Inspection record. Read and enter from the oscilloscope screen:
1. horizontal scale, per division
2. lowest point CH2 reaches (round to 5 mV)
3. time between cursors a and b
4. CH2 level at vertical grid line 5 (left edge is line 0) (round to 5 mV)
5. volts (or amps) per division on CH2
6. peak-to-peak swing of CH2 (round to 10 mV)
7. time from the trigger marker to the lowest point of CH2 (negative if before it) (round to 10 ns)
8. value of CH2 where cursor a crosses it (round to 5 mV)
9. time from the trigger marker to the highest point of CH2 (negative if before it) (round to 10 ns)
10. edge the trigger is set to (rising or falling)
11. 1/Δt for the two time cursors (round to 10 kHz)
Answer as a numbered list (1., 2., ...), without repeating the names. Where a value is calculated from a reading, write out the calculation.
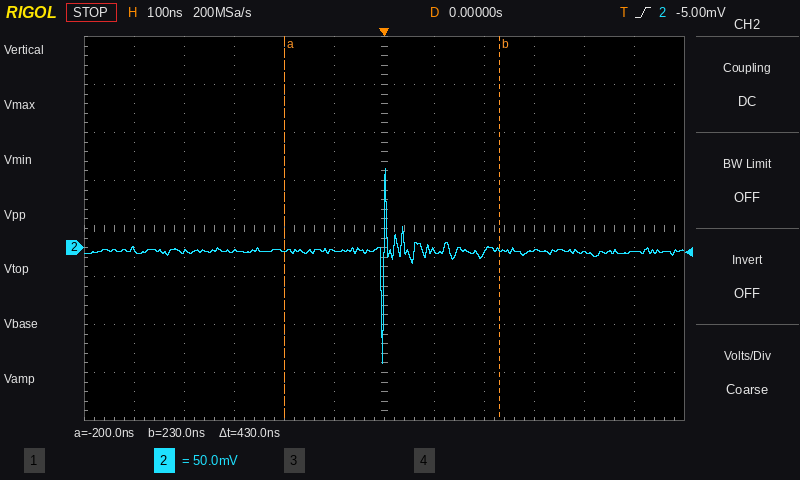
1. 100 ns
2. -120 mV
3. 430 ns
4. -5 mV
5. 50 mV
6. 200 mV
7. 0 ns
8. -5 mV
9. 0 ns
10. rising
11. 1 / 430 ns ≈ 2.33 MHz
